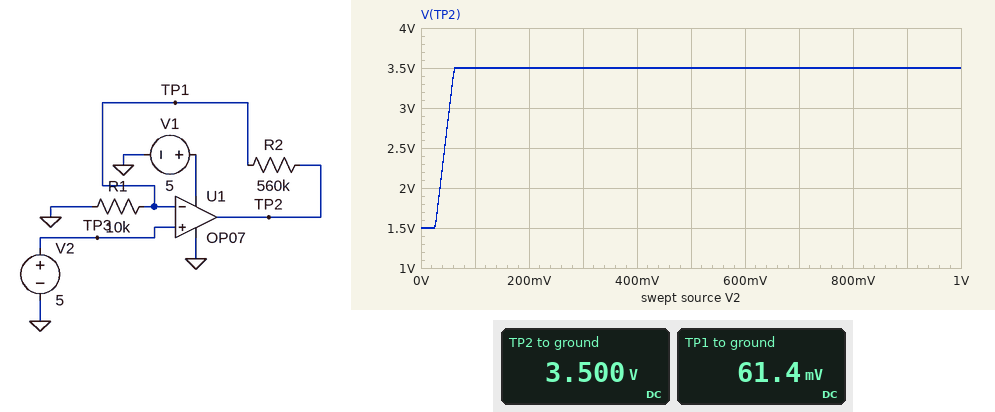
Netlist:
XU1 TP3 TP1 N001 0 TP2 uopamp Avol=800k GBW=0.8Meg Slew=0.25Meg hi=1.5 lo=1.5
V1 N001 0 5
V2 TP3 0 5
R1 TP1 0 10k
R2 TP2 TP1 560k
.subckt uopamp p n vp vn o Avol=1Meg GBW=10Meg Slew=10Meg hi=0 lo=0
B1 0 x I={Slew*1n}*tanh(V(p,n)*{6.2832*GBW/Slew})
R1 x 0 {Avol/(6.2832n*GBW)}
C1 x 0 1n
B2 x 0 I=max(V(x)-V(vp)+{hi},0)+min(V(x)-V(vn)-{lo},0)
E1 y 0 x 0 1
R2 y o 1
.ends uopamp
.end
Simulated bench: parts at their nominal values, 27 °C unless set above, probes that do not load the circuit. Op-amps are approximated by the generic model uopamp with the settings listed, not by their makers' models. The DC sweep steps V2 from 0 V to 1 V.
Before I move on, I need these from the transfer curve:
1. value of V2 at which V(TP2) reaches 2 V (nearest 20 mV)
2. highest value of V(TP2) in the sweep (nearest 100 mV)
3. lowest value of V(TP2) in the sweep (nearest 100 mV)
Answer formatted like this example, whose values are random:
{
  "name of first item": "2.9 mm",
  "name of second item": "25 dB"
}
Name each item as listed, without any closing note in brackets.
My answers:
{
  "value of V2 at which V(TP2) reaches 2 V": "40 mV",
  "highest value of V(TP2) in the sweep": "3.5 V",
  "lowest value of V(TP2) in the sweep": "1.5 V"
}
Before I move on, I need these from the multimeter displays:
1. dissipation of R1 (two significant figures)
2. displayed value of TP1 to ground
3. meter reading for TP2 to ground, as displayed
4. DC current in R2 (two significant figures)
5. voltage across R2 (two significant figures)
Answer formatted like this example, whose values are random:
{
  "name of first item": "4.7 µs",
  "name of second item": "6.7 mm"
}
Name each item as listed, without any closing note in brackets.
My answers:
{
  "dissipation of R1": "380 nW",
  "displayed value of TP1 to ground": "61.4 mV",
  "meter reading for TP2 to ground, as displayed": "3.500 V",
  "DC current in R2": "6.1 µA",
  "voltage across R2": "3.4 V"
}
